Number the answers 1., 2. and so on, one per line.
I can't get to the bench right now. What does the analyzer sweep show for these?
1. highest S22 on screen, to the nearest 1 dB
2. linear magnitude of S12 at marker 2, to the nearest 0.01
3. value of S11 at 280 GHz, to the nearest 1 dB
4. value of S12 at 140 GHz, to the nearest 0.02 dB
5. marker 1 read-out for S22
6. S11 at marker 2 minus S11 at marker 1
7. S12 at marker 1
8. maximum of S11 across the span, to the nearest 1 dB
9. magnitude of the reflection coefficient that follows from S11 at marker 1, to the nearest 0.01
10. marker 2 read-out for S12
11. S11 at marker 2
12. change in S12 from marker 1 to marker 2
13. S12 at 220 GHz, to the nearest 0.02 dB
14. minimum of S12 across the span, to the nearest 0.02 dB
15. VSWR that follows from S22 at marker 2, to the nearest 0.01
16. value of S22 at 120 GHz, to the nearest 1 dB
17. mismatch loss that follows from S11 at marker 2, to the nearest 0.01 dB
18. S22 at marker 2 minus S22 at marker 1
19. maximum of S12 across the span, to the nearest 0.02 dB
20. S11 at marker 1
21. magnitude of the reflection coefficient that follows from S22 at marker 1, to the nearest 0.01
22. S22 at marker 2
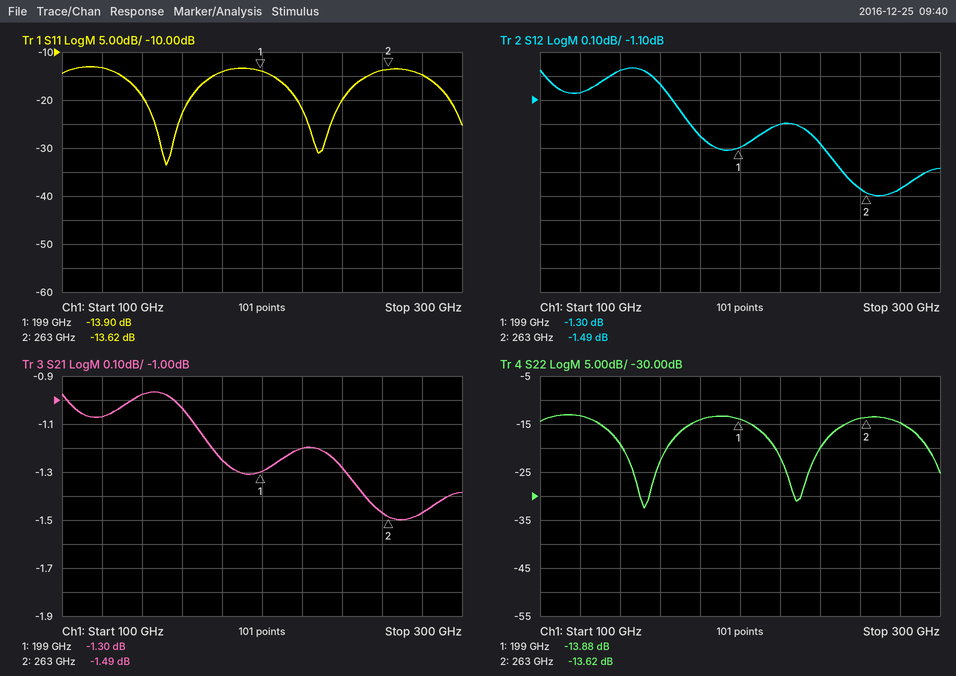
1. -13 dB
2. 0.84
3. -15 dB
4. -0.98 dB
5. -13.88 dB
6. 0.28 dB
7. -1.30 dB
8. -13 dB
9. 0.20
10. -1.49 dB
11. -13.62 dB
12. -0.19 dB
13. -1.20 dB
14. -1.50 dB
15. 1.53
16. -13 dB
17. 0.19 dB
18. 0.26 dB
19. -0.96 dB
20. -13.90 dB
21. 0.20
22. -13.62 dB
